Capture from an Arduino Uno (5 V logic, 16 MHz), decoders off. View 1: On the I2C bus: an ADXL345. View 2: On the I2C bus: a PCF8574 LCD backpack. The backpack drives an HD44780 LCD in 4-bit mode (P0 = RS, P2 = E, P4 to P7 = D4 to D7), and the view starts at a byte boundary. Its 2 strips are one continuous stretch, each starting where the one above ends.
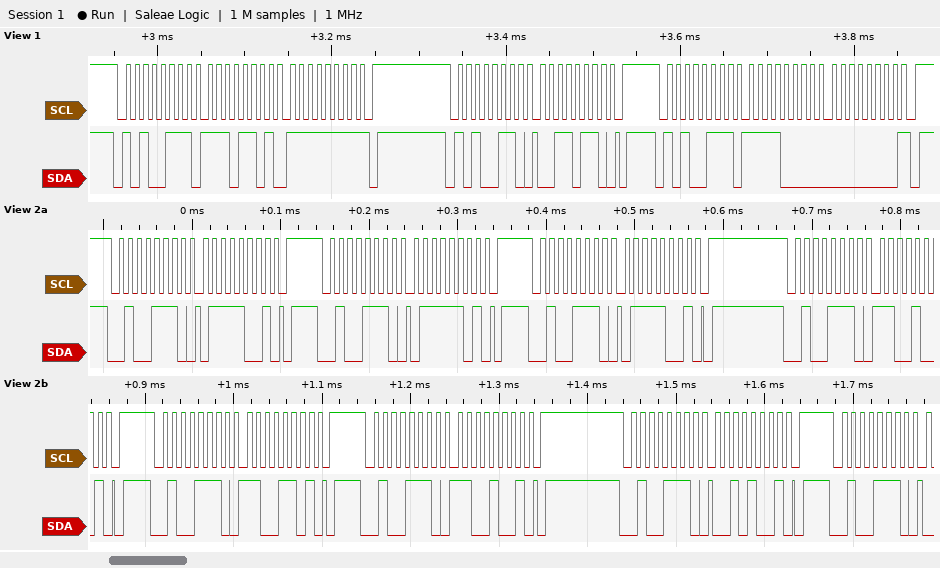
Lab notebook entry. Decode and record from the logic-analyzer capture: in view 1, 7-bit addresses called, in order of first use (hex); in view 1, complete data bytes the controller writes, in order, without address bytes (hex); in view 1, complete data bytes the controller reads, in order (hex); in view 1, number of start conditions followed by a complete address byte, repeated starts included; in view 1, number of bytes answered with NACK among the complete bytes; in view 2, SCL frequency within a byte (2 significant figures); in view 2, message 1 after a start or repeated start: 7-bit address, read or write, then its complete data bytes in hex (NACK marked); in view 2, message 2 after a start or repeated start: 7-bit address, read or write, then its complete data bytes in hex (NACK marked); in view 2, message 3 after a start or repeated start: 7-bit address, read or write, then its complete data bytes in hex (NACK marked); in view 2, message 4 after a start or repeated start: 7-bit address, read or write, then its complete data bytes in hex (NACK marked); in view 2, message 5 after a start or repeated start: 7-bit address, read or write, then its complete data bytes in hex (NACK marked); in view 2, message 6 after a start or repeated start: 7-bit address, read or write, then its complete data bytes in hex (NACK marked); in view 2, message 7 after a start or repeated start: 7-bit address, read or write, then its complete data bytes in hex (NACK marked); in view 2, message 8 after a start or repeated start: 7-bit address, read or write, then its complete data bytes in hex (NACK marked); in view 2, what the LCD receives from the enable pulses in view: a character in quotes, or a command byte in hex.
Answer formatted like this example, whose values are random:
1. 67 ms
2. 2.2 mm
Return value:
1. 0x53
2. 36
3. ED FF F0 00
4. 3
5. 2
6. 100 kHz
7. 0x27 write: 79
8. 0x27 write: 7D
9. 0x27 write: 79
10. 0x27 write: C9
11. 0x27 write: CD
12. 0x27 write: C9
13. 0x27 write: 29
14. 0x27 write
15. '|'
